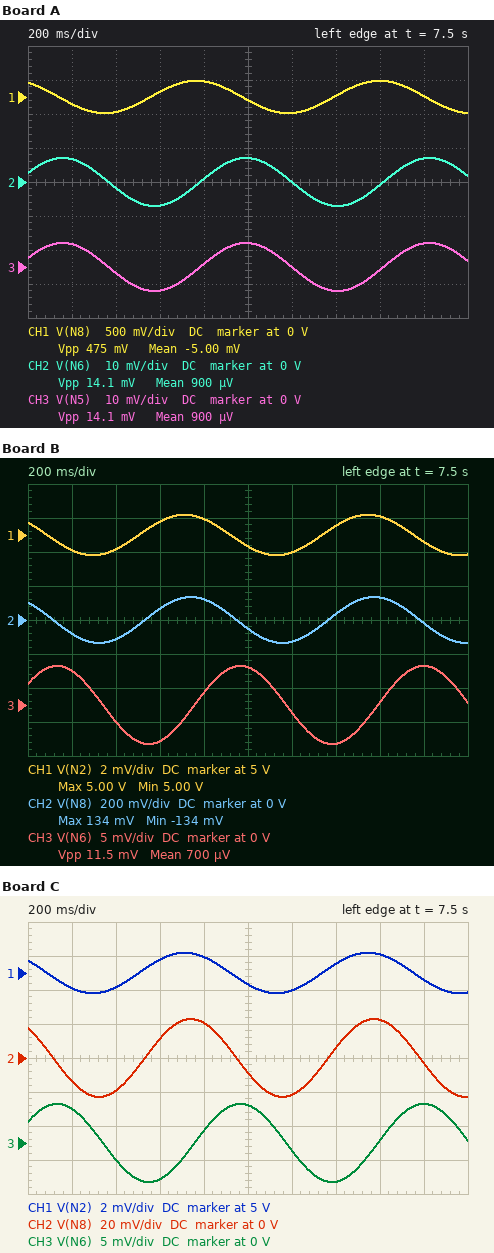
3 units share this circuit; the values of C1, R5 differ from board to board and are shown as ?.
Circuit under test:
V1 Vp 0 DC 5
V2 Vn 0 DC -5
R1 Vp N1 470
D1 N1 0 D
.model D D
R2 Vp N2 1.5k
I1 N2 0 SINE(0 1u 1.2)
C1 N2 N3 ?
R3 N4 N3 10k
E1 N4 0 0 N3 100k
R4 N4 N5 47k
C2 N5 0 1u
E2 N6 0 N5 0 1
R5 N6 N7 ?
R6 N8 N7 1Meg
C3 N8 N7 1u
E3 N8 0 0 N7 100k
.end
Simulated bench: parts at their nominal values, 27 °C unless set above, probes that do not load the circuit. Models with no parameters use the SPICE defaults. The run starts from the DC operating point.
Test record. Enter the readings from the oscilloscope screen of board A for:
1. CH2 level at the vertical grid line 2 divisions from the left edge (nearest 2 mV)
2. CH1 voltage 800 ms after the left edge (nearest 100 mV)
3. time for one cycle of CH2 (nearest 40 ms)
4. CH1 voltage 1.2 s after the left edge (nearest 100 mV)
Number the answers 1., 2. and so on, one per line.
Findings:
1. -2 mV
2. 200 mV
3. 840 ms
4. -200 mV
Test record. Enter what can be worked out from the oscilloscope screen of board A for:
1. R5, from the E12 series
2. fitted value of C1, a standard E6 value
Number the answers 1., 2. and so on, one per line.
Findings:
1. 3.9 kΩ
2. 100 µF
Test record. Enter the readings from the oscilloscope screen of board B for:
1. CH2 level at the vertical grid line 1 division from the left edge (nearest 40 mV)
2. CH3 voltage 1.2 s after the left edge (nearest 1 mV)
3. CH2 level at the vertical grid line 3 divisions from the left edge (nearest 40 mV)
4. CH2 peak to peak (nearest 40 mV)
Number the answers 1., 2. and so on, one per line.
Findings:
1. -80 mV
2. -1 mV
3. 80 mV
4. 280 mV
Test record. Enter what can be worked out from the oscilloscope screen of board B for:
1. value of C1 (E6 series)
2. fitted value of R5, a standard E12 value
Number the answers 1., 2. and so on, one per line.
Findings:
1. 68 µF
2. 5.6 kΩ
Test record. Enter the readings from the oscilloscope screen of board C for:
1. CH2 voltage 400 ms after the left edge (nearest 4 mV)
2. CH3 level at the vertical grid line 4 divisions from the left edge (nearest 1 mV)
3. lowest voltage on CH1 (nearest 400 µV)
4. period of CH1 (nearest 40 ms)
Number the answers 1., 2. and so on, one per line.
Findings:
1. -20 mV
2. 2 mV
3. 4.9988 V
4. 840 ms
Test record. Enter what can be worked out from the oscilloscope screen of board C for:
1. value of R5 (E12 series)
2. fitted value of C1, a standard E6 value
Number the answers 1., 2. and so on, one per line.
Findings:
1. 33 kΩ
2. 68 µF
